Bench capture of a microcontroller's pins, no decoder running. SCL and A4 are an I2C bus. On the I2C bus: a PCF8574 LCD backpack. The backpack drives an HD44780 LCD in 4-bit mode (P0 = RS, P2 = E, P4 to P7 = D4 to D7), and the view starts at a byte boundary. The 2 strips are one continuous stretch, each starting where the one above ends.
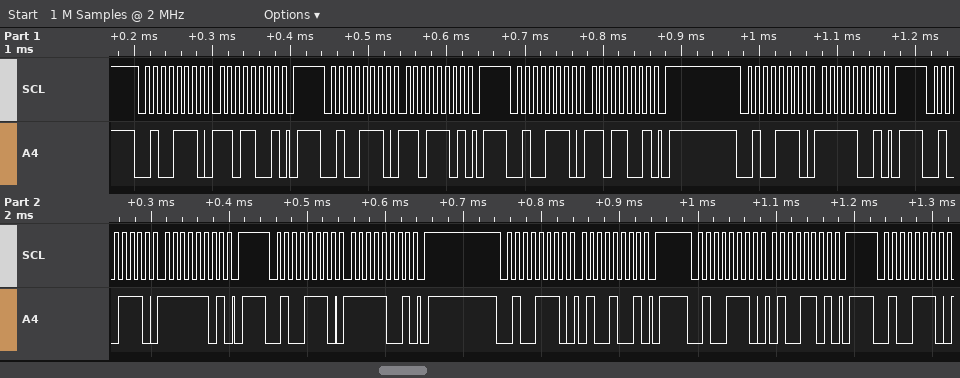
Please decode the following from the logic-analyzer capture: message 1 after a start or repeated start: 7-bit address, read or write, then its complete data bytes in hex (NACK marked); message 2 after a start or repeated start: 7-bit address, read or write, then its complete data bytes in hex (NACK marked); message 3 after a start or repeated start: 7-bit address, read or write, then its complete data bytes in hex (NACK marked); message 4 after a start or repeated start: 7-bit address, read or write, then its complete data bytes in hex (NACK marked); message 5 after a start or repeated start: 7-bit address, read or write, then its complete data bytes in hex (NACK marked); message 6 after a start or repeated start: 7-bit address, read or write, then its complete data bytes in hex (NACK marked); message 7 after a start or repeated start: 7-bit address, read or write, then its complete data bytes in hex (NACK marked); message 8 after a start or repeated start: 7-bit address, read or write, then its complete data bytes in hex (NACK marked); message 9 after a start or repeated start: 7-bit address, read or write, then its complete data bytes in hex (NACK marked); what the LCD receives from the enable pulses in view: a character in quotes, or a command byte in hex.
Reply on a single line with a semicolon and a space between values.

0x27 write: D9; 0x27 write: DD; 0x27 write: D9; 0x27 write: F9; 0x27 write: FD; 0x27 write: F9; 0x27 write: 49; 0x27 write: 4D; 0x27 write; data 0xDF
